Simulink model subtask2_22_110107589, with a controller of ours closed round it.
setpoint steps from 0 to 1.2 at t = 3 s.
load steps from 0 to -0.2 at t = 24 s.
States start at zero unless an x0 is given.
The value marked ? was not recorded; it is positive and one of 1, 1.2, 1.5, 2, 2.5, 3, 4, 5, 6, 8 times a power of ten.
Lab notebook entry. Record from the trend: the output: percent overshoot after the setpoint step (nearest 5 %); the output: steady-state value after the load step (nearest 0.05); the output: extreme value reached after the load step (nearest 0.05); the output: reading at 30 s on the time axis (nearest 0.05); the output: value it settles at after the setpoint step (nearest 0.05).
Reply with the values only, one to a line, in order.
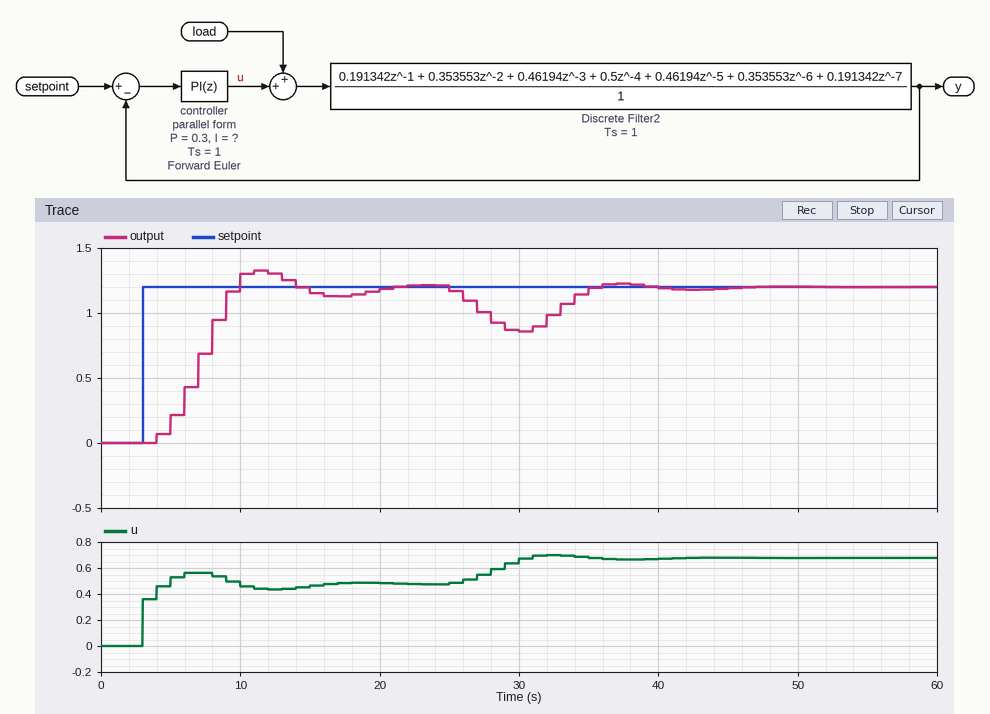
10 %
1.20
0.85
0.85
1.20
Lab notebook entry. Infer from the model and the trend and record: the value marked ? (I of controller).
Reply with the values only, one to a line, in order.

0.1
